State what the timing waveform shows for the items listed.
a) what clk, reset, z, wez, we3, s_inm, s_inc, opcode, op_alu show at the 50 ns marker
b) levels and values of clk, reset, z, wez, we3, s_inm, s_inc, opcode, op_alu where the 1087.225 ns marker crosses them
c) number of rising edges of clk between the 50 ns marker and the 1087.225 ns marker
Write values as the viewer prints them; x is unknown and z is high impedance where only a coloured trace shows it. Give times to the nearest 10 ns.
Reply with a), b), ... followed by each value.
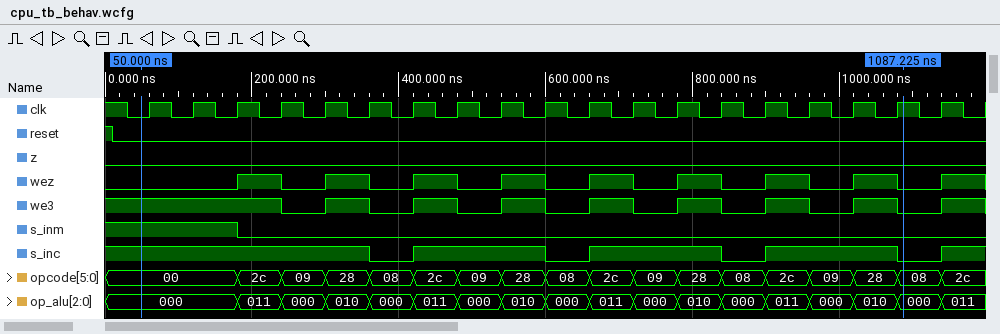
a) clk=0, reset=0, z=0, wez=0, we3=1, s_inm=1, s_inc=1, opcode=00, op_alu=000
b) clk=1, reset=0, z=0, wez=0, we3=0, s_inm=0, s_inc=0, opcode=08, op_alu=000
c) 18
